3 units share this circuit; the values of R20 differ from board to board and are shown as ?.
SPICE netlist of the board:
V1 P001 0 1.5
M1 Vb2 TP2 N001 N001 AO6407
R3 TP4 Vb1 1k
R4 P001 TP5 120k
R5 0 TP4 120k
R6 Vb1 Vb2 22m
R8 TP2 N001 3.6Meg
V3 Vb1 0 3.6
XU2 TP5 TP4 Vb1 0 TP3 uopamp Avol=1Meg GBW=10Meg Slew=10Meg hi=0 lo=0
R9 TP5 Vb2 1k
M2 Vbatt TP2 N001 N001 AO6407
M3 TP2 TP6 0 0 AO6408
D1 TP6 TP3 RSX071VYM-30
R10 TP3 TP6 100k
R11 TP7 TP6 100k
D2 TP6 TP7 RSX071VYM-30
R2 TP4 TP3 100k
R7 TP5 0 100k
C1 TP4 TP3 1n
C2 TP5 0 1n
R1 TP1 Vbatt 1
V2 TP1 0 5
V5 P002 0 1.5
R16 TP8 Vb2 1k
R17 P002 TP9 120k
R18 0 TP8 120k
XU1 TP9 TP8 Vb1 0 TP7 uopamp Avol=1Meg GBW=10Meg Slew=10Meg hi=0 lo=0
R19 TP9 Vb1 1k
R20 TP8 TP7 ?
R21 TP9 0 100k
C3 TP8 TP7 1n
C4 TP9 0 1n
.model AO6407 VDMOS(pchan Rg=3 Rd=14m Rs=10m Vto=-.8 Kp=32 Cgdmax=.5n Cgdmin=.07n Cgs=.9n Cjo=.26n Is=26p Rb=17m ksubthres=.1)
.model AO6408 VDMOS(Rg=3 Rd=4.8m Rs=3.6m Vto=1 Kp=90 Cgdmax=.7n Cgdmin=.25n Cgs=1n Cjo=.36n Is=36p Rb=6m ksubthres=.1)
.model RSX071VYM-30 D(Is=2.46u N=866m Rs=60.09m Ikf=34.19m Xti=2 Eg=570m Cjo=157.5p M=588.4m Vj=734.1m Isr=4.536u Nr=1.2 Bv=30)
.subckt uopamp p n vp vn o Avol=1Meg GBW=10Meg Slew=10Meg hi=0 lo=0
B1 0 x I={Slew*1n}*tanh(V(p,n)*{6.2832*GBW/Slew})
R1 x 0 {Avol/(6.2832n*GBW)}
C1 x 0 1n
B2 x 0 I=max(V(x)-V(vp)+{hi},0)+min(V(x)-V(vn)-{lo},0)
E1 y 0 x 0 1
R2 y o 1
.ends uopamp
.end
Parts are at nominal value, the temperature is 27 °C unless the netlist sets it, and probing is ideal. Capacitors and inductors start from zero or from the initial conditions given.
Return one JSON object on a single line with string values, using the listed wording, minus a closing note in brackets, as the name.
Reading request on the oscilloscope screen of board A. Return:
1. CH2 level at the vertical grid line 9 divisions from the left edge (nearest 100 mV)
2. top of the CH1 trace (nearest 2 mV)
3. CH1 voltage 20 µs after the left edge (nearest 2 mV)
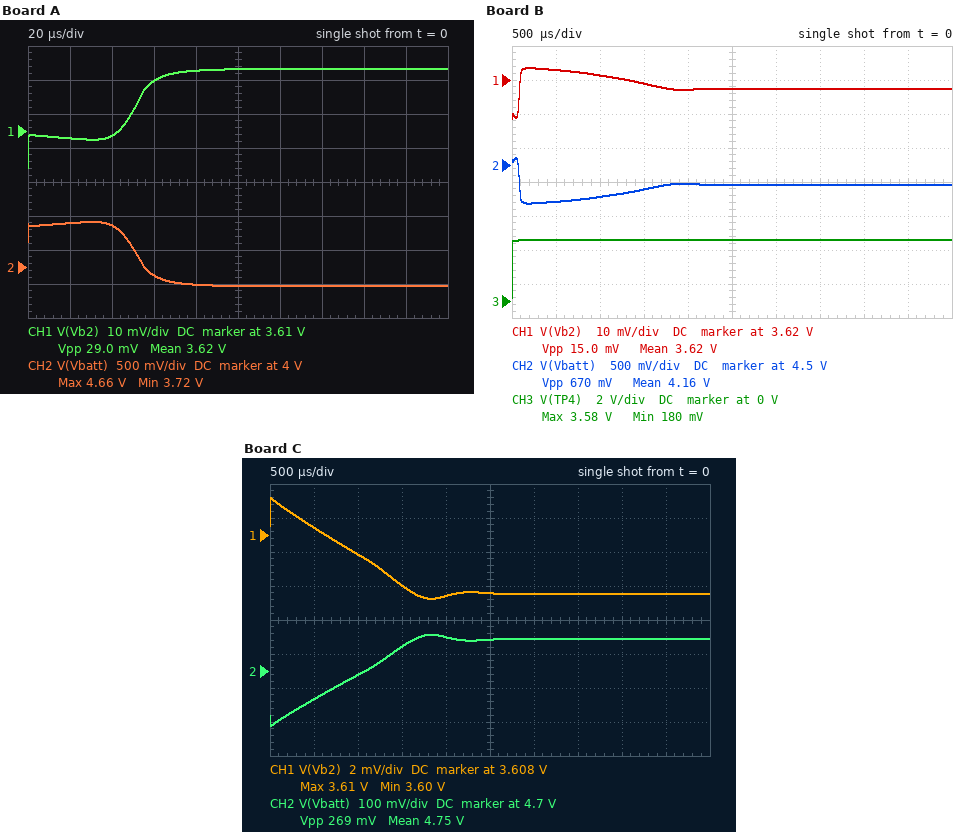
{"CH2 level at the vertical grid line 9 divisions from the left edge": "3.7 V", "top of the CH1 trace": "3.628 V", "CH1 voltage 20 µs after the left edge": "3.608 V"}
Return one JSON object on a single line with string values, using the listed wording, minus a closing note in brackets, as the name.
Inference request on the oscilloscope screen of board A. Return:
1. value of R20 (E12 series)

{"value of R20": "39 kΩ"}
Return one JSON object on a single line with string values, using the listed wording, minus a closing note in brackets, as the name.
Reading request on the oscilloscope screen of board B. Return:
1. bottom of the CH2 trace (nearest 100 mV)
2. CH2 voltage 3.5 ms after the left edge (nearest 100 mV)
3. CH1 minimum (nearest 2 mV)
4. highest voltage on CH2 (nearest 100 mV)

{"bottom of the CH2 trace": "3.9 V", "CH2 voltage 3.5 ms after the left edge": "4.2 V", "CH1 minimum": "3.608 V", "highest voltage on CH2": "4.6 V"}
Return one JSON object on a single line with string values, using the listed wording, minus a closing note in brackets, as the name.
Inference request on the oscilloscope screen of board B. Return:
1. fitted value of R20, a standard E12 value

{"fitted value of R20, a standard E12 value": "82 kΩ"}
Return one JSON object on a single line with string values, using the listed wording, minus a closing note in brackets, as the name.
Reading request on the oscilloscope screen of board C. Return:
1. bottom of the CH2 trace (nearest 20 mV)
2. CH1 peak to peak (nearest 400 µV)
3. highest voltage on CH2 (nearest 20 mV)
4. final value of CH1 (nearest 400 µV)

{"bottom of the CH2 trace": "4.54 V", "CH1 peak to peak": "6.0 mV", "highest voltage on CH2": "4.80 V", "final value of CH1": "3.6044 V"}
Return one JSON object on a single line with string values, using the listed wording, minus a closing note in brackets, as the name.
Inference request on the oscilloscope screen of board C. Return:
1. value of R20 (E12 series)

{"value of R20": "120 kΩ"}
